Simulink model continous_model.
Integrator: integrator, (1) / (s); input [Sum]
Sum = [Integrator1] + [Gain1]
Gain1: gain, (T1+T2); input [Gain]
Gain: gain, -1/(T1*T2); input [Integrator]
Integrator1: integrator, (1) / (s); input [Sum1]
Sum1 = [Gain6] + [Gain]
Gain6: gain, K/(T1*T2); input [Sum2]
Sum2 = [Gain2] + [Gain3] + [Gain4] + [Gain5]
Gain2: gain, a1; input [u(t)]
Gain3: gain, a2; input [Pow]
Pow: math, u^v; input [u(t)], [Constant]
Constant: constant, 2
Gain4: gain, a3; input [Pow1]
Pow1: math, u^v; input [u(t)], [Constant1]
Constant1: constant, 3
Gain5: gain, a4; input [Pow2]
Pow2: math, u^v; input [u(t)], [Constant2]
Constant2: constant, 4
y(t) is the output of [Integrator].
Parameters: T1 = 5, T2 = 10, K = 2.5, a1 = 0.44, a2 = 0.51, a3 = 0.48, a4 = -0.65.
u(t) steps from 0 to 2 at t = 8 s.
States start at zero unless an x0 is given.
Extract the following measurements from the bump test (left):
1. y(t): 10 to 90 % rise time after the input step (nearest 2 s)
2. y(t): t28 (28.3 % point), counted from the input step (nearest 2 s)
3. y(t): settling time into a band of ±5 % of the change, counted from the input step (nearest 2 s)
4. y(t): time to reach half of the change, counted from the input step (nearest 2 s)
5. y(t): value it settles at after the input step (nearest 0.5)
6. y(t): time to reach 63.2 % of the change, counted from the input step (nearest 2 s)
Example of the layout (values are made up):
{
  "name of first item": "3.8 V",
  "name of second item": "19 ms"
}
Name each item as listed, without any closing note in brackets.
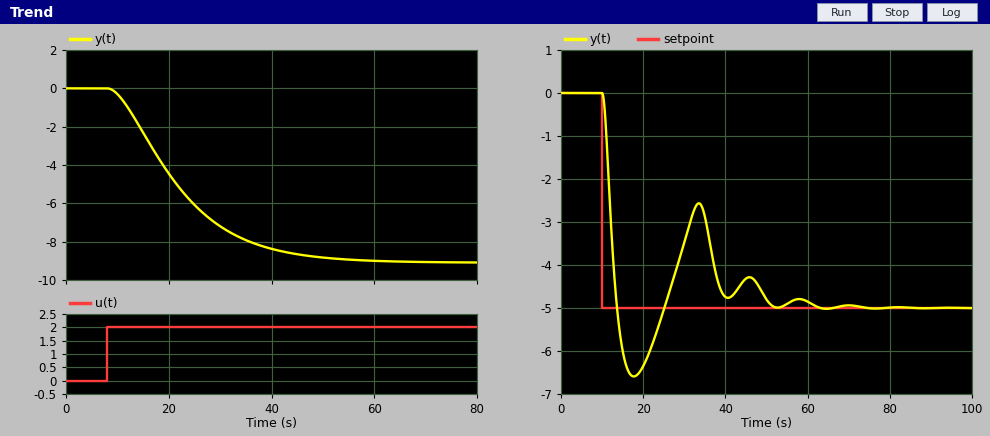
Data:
{
  "y(t): 10 to 90 % rise time after the input step": "26 s",
  "y(t): t28 (28.3 % point), counted from the input step": "8 s",
  "y(t): settling time into a band of ±5 % of the change, counted from the input step": "36 s",
  "y(t): time to reach half of the change, counted from the input step": "12 s",
  "y(t): value it settles at after the input step": "-9.0",
  "y(t): time to reach 63.2 % of the change, counted from the input step": "16 s"
}
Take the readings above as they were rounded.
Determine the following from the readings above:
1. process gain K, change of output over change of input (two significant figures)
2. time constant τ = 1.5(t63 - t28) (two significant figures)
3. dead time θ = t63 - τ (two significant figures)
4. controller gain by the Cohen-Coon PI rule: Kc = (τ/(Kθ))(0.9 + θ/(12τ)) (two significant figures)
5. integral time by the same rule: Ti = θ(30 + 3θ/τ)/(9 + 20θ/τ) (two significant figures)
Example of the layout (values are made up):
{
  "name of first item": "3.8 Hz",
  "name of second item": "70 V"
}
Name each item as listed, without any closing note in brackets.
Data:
{
  "process gain K, change of output over change of input": "-4.5",
  "time constant τ = 1.5(t63 - t28)": "12 s",
  "dead time θ = t63 - τ": "4.0 s",
  "controller gain by the Cohen-Coon PI rule: Kc = (τ/(Kθ))(0.9 + θ/(12τ))": "-0.62",
  "integral time by the same rule: Ti = θ(30 + 3θ/τ)/(9 + 20θ/τ)": "7.9 s"
}
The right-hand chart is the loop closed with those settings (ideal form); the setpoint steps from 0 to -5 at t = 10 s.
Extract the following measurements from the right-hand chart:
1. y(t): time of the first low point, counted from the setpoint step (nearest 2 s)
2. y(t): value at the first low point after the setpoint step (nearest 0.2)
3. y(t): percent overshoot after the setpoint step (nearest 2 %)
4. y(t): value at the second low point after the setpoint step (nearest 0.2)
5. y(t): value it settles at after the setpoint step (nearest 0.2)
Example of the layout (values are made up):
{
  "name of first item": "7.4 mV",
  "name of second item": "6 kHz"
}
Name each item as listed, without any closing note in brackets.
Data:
{
  "y(t): time of the first low point, counted from the setpoint step": "8 s",
  "y(t): value at the first low point after the setpoint step": "-6.6",
  "y(t): percent overshoot after the setpoint step": "32 %",
  "y(t): value at the second low point after the setpoint step": "-4.8",
  "y(t): value it settles at after the setpoint step": "-5.0"
}
